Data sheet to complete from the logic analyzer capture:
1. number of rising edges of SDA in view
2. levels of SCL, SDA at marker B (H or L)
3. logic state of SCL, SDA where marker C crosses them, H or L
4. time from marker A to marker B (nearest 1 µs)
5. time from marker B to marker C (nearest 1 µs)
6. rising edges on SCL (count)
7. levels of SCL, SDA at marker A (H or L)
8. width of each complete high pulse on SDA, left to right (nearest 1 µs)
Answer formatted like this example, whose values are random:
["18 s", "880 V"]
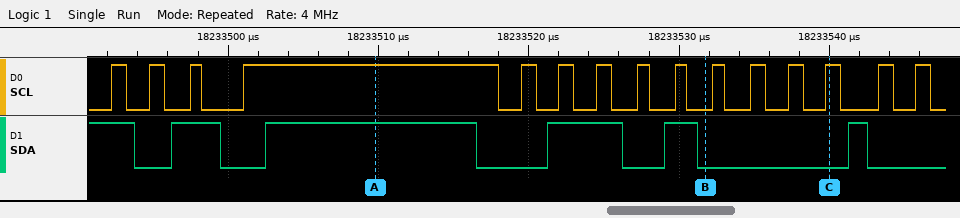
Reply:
["5", "SCL=L, SDA=L", "SCL=H, SDA=L", "22 µs", "8 µs", "15", "SCL=H, SDA=H", "3 µs, 14 µs, 5 µs, 2 µs, 1 µs"]
